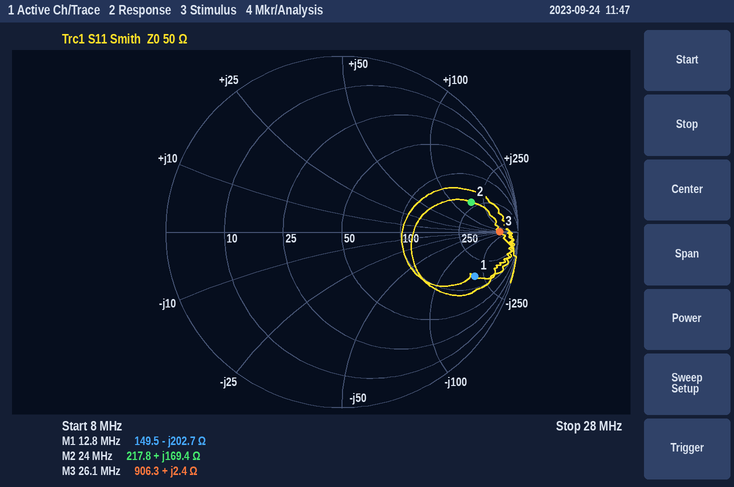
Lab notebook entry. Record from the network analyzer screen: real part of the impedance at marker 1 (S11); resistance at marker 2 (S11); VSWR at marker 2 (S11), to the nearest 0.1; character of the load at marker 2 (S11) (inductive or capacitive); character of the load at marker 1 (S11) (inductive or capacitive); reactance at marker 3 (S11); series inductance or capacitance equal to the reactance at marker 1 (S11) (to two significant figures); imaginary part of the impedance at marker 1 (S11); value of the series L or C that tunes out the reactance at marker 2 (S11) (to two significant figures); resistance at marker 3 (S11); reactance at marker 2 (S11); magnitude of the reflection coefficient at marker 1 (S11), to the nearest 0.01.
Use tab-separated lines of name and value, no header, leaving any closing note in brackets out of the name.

real part of the impedance at marker 1	149.5 Ω
resistance at marker 2	217.8 Ω
VSWR at marker 2 (S11), to the nearest 0.1	7.1
character of the load at marker 2 (S11)	inductive
character of the load at marker 1 (S11)	capacitive
reactance at marker 3	+2.4 Ω
series inductance or capacitance equal to the reactance at marker 1 (S11)	61 pF
imaginary part of the impedance at marker 1	-202.7 Ω
value of the series L or C that tunes out the reactance at marker 2 (S11)	39 pF
resistance at marker 3	906.3 Ω
reactance at marker 2	+169.4 Ω
magnitude of the reflection coefficient at marker 1 (S11), to the nearest 0.01	0.79
